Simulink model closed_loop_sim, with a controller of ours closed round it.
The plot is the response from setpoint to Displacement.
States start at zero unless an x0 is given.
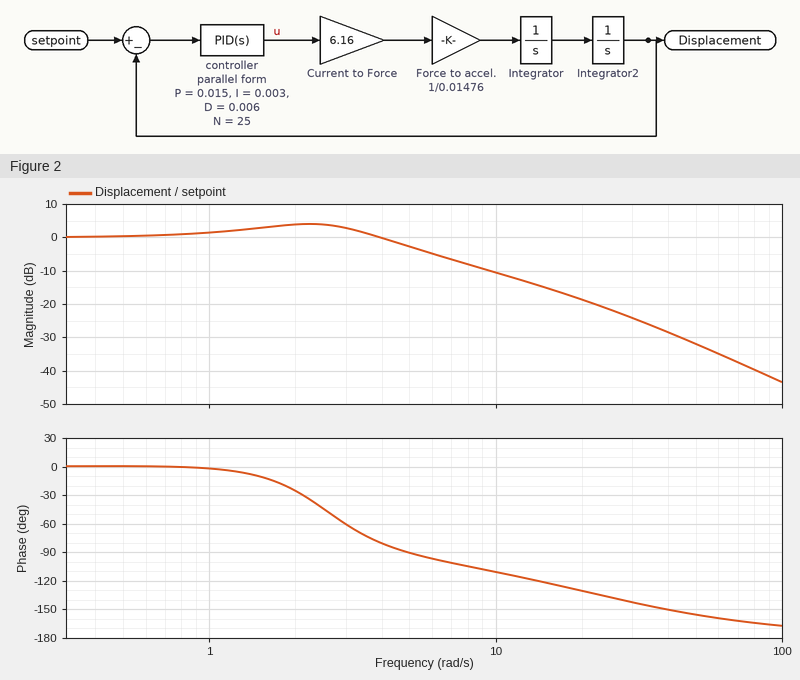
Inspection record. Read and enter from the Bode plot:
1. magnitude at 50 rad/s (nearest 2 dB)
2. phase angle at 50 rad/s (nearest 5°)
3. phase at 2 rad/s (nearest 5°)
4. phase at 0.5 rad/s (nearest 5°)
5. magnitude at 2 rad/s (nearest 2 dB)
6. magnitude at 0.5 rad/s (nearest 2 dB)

-32 dB
-155°
-25°
0°
4 dB
0 dB
